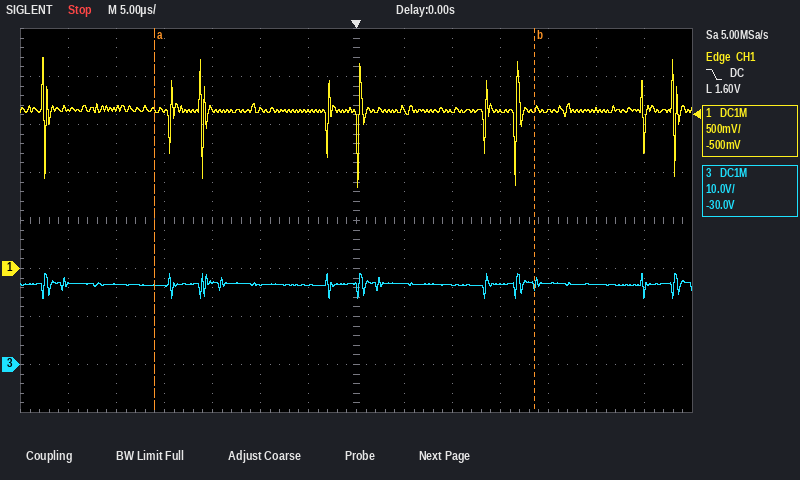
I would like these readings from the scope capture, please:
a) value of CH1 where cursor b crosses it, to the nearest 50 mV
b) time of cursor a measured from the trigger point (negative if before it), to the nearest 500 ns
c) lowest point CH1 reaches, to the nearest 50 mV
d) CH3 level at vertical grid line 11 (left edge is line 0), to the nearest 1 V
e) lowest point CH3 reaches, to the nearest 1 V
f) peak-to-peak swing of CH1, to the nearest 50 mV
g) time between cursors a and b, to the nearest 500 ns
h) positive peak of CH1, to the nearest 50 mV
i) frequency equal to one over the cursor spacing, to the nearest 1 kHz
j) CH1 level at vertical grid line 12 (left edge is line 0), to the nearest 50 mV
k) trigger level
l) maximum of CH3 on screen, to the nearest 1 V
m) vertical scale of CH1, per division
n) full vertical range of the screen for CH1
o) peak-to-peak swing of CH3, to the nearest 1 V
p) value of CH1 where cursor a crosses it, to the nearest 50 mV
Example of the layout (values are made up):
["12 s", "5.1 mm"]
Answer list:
["1.65 V", "-21.0 µs", "850 mV", "17 V", "14 V", "1.35 V", "39.5 µs", "2.20 V", "25 kHz", "1.65 V", "1.60 V", "19 V", "500 mV", "4 V", "5 V", "1.65 V"]
